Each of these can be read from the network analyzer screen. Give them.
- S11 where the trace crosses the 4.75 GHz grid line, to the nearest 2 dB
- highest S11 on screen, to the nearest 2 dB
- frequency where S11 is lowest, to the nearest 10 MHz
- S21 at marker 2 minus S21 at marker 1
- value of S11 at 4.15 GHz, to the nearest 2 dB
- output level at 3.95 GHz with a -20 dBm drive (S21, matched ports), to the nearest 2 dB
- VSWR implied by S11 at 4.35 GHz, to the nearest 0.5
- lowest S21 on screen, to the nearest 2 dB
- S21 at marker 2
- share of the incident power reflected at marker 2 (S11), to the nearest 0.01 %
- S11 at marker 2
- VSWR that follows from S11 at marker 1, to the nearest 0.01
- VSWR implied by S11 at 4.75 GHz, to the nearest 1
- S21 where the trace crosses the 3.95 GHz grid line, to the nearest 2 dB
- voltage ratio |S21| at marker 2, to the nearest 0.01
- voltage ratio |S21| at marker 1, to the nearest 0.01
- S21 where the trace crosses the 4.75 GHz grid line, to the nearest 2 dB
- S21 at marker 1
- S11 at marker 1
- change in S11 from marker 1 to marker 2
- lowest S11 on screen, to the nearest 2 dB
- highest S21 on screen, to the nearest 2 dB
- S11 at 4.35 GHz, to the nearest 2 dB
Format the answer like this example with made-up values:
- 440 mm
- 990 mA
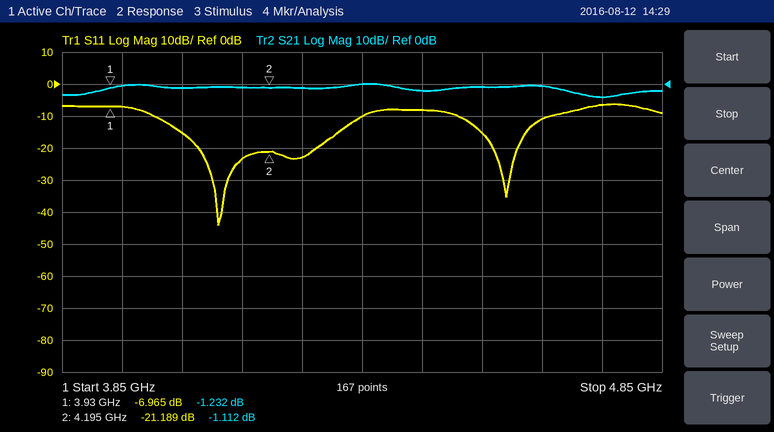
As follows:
- -6 dB
- -6 dB
- 4.11 GHz
- 0.120 dB
- -24 dB
- -20 dBm
- 2.0
- -4 dB
- -1.112 dB
- 0.76 %
- -21.189 dB
- 2.63
- 3
- 0 dB
- 0.88
- 0.87
- -4 dB
- -1.232 dB
- -6.965 dB
- -14.224 dB
- -44 dB
- 0 dB
- -10 dB
